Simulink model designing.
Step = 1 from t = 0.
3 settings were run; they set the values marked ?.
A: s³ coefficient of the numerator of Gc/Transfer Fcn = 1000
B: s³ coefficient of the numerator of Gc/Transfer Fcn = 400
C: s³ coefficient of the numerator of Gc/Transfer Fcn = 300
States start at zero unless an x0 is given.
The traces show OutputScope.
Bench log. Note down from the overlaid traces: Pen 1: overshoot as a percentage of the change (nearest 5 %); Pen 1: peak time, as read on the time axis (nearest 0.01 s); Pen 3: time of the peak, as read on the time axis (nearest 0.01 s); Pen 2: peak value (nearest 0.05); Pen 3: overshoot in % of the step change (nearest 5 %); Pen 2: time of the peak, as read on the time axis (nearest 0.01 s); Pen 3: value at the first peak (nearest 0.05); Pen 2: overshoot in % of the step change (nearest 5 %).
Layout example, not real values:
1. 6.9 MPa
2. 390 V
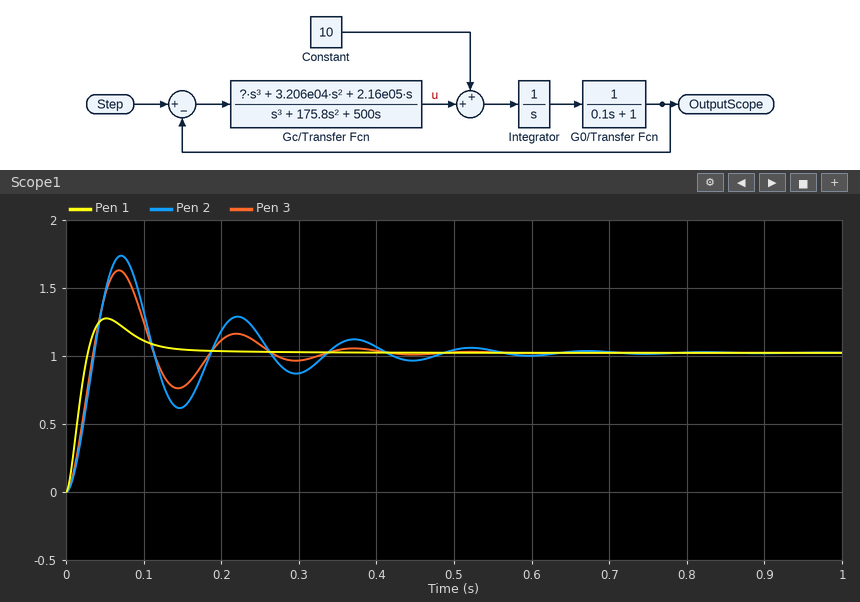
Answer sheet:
1. 25 %
2. 0.05 s
3. 0.07 s
4. 1.75
5. 60 %
6. 0.07 s
7. 1.65
8. 70 %
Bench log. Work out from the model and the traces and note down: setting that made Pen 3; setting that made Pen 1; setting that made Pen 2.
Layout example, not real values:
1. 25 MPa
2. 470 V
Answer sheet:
1. B
2. A
3. C
